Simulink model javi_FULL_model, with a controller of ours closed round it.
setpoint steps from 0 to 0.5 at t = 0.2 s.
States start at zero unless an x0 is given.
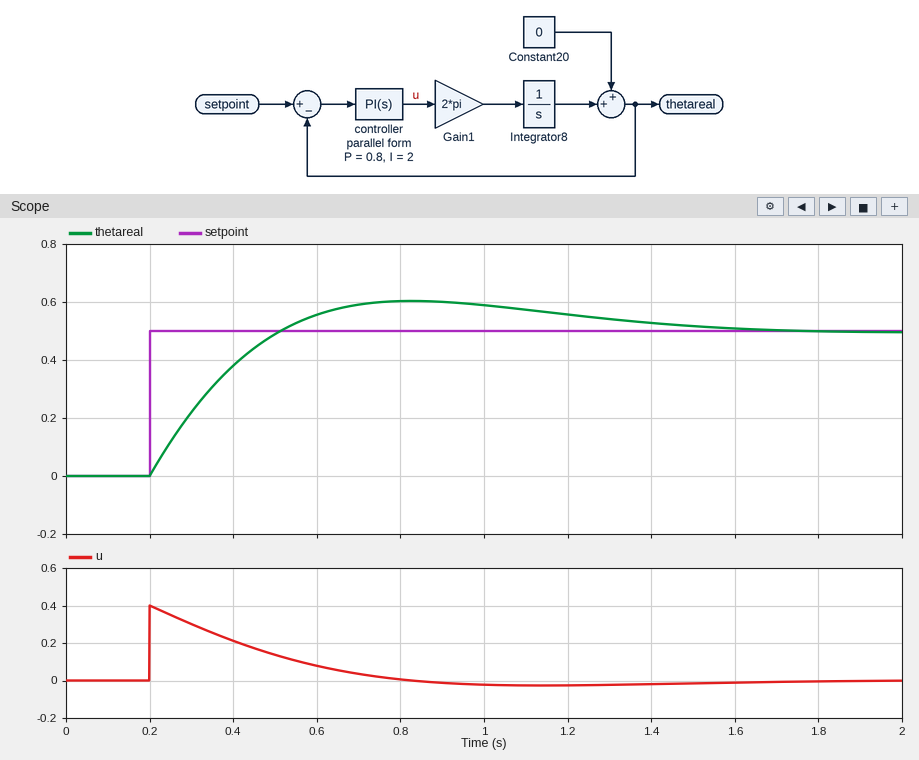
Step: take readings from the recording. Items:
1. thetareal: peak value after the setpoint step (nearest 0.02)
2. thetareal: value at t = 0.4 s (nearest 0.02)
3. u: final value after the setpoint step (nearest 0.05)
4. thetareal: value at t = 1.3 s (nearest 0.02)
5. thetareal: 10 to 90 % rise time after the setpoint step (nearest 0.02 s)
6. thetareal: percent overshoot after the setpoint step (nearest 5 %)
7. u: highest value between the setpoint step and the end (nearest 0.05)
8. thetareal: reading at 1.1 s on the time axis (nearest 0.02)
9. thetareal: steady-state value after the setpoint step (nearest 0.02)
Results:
0.60
0.38
0.00
0.54
0.24 s
20 %
0.40
0.58
0.50
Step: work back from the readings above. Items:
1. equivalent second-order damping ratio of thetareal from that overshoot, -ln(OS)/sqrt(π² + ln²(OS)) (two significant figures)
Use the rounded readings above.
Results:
0.46
